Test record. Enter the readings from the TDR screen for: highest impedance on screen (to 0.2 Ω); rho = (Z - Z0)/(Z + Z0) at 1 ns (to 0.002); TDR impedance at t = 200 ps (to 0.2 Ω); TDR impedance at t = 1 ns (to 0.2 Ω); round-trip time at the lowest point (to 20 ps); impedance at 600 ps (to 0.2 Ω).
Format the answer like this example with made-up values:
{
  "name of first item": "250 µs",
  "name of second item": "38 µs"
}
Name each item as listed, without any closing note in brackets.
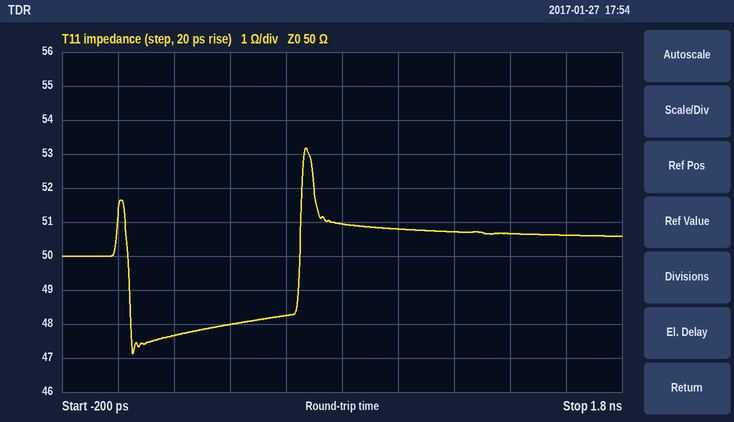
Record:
{
  "highest impedance on screen": "53.2 Ω",
  "rho = (Z - Z0)/(Z + Z0) at 1 ns": "+0.008",
  "TDR impedance at t = 200 ps": "47.6 Ω",
  "TDR impedance at t = 1 ns": "50.8 Ω",
  "round-trip time at the lowest point": "60 ps",
  "impedance at 600 ps": "48.2 Ω"
}
